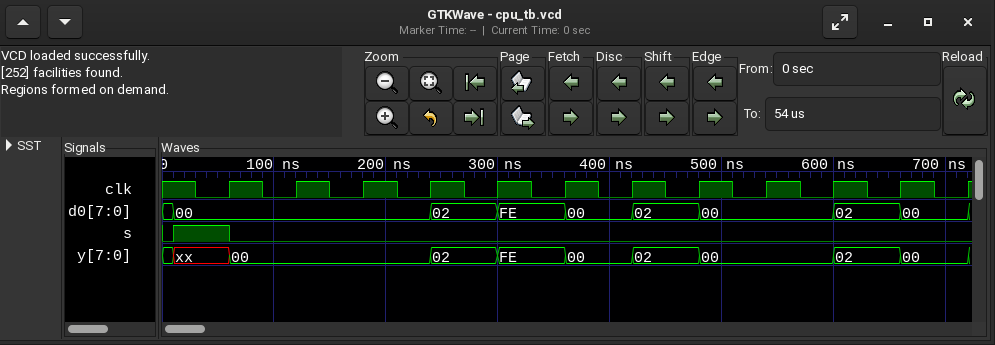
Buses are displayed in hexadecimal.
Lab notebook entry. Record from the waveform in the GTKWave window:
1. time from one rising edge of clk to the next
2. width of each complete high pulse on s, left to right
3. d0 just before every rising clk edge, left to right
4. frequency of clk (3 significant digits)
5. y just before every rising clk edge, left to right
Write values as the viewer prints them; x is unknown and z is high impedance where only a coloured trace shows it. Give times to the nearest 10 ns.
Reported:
60 ns
50 ns
00, 00, 00, 00, 02, FE, 00, 02, 00, 00, 02, 00
16.7 MHz
xx, 00, 00, 00, 02, FE, 00, 02, 00, 00, 02, 00
